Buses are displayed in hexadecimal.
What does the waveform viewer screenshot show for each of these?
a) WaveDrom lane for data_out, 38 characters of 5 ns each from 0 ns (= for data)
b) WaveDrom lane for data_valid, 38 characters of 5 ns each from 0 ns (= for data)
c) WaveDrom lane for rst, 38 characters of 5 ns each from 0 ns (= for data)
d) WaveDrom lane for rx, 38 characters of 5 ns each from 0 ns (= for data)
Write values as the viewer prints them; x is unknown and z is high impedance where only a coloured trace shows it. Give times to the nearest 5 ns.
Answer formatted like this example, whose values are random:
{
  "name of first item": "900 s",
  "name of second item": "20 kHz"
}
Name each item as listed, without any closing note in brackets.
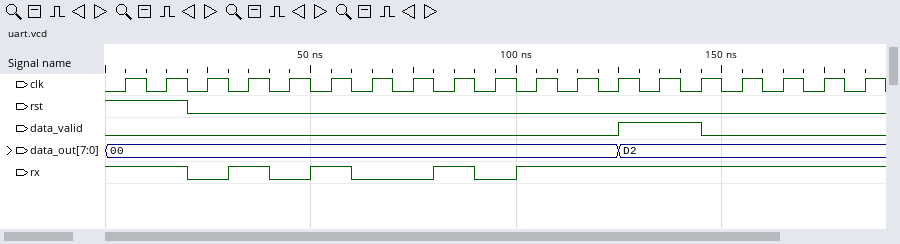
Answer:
{
  "WaveDrom lane for data_out, 38 characters of 5 ns each from 0 ns": "{name: 'data_out', wave: '=........................=............', data: '00 D2'}",
  "WaveDrom lane for data_valid, 38 characters of 5 ns each from 0 ns": "{name: 'data_valid', wave: '0........................1...0........'}",
  "WaveDrom lane for rst, 38 characters of 5 ns each from 0 ns": "{name: 'rst', wave: '1...0.................................'}",
  "WaveDrom lane for rx, 38 characters of 5 ns each from 0 ns": "{name: 'rx', wave: '1...0.1.0.1.0...1.0.1.................'}"
}
